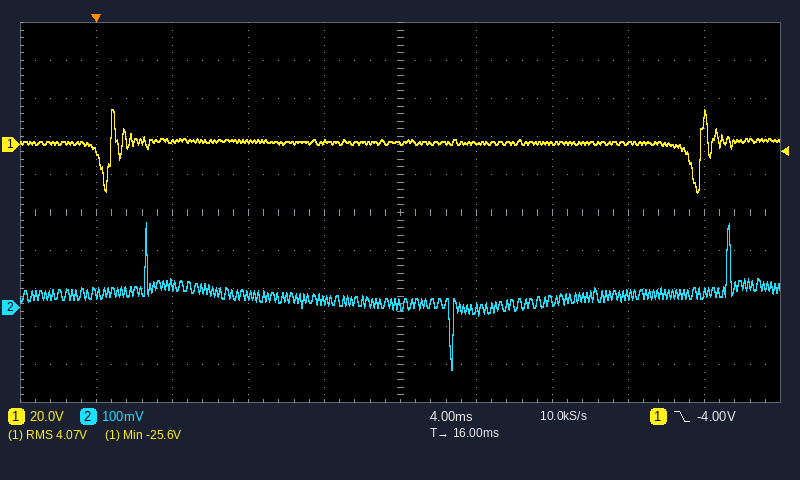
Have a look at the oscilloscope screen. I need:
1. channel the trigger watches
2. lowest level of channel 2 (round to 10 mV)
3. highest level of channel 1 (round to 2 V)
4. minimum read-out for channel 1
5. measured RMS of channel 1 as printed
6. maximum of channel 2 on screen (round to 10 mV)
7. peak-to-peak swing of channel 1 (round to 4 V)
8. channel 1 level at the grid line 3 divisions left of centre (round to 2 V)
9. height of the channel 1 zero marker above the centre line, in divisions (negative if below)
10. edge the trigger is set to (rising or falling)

channel 1
-160 mV
18 V
-25.6 V
4.07 V
220 mV
44 V
2 V
+1.8 div
falling
